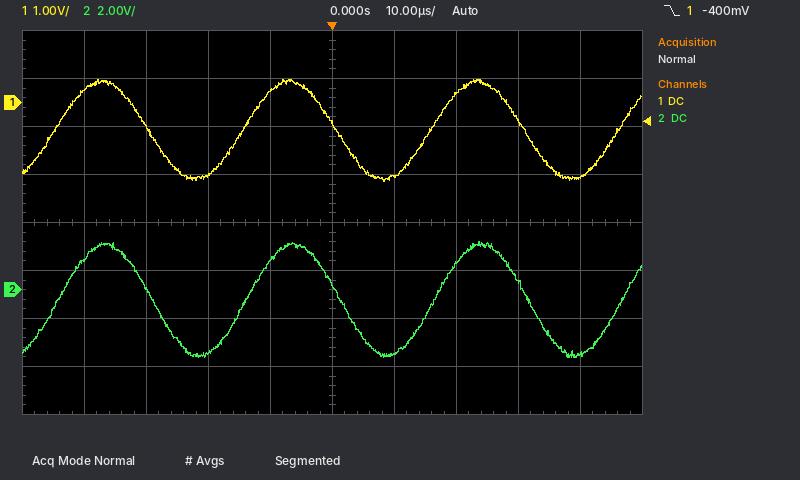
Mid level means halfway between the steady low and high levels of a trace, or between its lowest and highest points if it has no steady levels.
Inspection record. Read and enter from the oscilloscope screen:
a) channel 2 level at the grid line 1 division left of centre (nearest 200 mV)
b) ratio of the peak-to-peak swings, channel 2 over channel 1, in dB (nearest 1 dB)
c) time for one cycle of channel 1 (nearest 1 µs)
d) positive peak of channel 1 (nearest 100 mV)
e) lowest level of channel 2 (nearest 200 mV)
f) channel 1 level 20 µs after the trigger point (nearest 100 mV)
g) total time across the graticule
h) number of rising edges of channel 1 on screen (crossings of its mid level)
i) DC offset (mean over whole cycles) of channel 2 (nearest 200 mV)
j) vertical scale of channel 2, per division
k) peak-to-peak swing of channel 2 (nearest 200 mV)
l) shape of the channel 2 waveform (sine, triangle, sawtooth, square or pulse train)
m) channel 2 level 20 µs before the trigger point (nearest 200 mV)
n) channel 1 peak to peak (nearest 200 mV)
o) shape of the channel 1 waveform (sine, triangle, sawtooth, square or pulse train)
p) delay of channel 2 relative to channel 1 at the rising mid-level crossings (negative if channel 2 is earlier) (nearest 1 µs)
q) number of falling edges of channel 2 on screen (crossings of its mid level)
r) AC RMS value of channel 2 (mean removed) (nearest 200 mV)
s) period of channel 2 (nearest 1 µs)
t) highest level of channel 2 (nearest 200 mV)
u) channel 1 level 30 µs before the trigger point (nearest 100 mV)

1.2 V
7 dB
30 µs
500 mV
-2.8 V
200 mV
100 µs
4
-400 mV
2 V
4.8 V
sine
-2.6 V
2.2 V
sine
+1 µs
3
1.6 V
30 µs
2.0 V
-500 mV
